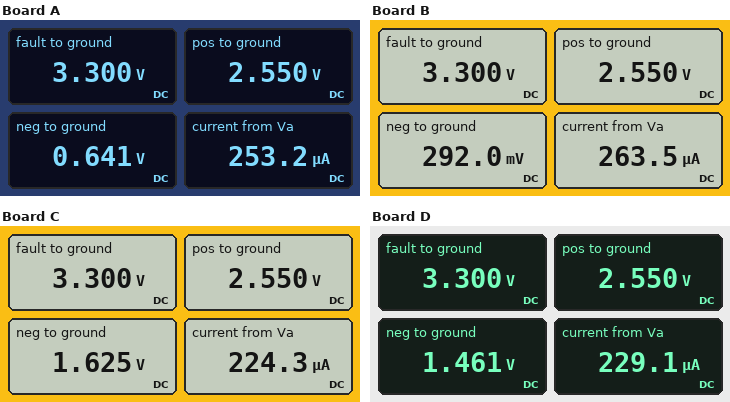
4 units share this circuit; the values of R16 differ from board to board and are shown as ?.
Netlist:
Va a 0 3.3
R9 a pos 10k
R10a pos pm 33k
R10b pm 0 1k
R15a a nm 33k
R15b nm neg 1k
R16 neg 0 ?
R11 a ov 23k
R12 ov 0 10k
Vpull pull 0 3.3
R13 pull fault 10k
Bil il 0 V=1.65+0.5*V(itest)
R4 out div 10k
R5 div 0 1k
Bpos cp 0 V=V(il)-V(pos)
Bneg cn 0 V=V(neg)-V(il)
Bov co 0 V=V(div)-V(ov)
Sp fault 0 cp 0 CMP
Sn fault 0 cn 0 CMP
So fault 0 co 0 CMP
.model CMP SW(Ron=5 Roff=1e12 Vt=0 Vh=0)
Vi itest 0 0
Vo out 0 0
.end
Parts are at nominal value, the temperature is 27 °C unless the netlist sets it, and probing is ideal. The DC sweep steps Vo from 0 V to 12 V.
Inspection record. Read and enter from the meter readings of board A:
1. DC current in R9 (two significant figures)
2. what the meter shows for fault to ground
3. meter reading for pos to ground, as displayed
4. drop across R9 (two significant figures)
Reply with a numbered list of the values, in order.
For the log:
1. 75 µA
2. 3.300 V
3. 2.550 V
4. 750 mV
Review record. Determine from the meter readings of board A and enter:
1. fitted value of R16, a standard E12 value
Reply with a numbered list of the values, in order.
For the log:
1. 8.2 kΩ
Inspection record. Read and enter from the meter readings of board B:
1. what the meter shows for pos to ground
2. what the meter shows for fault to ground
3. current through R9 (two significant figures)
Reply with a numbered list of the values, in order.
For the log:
1. 2.550 V
2. 3.300 V
3. 75 µA
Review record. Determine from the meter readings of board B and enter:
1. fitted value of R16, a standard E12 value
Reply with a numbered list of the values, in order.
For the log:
1. 3.3 kΩ
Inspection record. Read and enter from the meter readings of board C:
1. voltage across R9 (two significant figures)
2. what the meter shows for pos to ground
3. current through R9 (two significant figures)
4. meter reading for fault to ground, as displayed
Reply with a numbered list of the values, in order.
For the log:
1. 750 mV
2. 2.550 V
3. 75 µA
4. 3.300 V
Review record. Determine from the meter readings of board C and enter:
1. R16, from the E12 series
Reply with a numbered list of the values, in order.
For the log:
1. 33 kΩ
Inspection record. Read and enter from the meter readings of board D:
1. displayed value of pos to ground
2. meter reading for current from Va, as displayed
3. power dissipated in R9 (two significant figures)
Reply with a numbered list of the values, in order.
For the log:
1. 2.550 V
2. 229.1 µA
3. 56 µW
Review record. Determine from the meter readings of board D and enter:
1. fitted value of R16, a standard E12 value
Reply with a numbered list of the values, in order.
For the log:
1. 27 kΩ
